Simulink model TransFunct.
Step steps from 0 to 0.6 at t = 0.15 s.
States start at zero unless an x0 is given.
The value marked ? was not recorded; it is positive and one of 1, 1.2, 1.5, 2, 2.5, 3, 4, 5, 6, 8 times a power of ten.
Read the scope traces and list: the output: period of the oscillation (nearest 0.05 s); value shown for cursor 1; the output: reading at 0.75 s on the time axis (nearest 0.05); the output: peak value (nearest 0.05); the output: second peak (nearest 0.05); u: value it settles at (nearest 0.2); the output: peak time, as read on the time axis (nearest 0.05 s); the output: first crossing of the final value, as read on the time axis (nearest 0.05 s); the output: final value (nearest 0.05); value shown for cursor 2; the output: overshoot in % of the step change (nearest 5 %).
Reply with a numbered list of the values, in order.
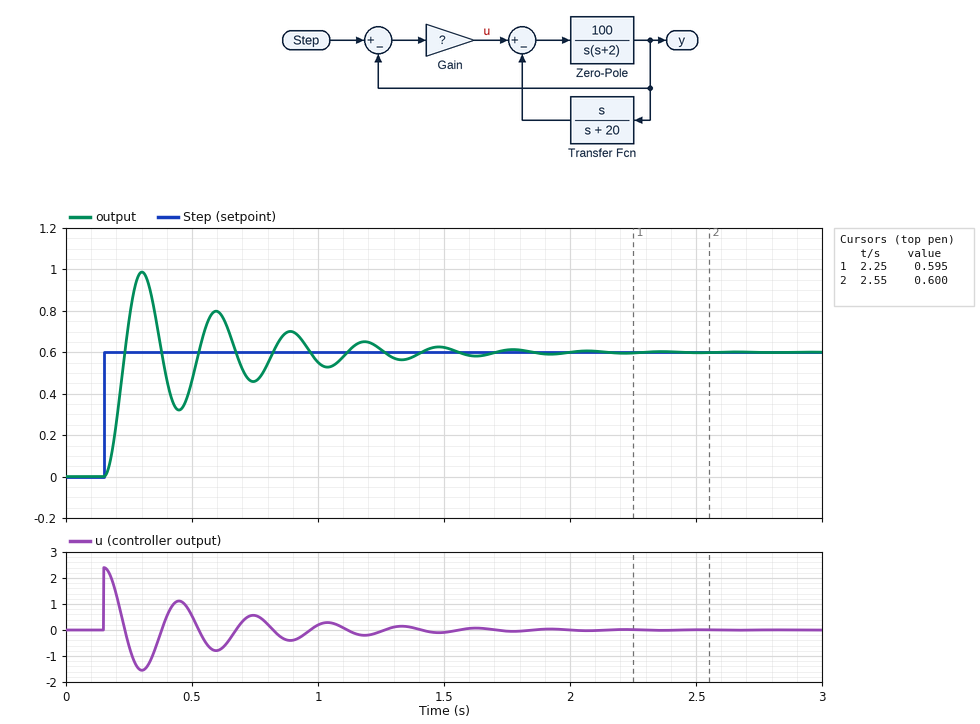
1. 0.30 s
2. 0.595
3. 0.45
4. 1.00
5. 0.80
6. 0.0
7. 0.30 s
8. 0.25 s
9. 0.60
10. 0.600
11. 65 %
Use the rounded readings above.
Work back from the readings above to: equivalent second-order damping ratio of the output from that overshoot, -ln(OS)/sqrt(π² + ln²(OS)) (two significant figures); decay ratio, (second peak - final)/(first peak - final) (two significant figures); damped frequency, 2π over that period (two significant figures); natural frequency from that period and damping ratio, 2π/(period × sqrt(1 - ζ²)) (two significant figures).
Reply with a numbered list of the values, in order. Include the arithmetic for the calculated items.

1. ln(0.65) = -0.431; 0.431 / sqrt(9.870 + 0.186) = 0.14
2. (0.8 - 0.6) / (1 - 0.6) = 0.50
3. 2π / 0.3 = 21 rad/s
4. 2π / (0.3 × sqrt(1 - 0.14²)) = 21 rad/s
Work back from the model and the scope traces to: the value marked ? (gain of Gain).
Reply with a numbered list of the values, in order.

1. 4
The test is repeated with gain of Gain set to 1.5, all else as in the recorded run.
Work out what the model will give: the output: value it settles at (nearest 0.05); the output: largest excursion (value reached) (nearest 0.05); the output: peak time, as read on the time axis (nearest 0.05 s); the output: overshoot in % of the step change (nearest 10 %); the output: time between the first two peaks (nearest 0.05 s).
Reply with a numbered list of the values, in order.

1. 0.60
2. 0.85
3. 0.40 s
4. 40 %
5. 0.45 s
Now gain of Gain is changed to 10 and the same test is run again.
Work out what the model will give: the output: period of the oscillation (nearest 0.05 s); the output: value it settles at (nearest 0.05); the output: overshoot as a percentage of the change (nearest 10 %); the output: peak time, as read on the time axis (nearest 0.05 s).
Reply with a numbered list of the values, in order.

1. 0.20 s
2. 0.60
3. 80 %
4. 0.25 s
